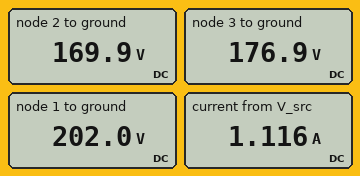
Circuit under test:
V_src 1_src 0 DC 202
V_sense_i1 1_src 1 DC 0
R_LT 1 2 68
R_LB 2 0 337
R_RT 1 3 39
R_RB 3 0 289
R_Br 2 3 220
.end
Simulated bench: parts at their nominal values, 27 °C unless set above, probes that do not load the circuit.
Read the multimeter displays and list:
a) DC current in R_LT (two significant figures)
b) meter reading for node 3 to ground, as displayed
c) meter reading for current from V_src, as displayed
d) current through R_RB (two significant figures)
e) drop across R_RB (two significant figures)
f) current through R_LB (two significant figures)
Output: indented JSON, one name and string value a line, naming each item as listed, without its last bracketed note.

{
  "DC current in R_LT": "470 mA",
  "meter reading for node 3 to ground, as displayed": "176.9 V",
  "meter reading for current from V_src, as displayed": "1.116 A",
  "current through R_RB": "610 mA",
  "drop across R_RB": "180 V",
  "current through R_LB": "500 mA"
}
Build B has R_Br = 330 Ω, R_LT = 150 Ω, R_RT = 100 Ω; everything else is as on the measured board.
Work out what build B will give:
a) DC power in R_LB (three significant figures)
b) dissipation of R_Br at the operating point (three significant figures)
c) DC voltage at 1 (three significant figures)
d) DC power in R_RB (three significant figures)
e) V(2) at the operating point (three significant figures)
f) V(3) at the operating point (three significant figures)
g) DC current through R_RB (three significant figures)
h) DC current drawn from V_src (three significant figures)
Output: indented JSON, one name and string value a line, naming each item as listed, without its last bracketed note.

{
  "DC power in R_LB": "59.7 W",
  "dissipation of R_Br at the operating point": "135 mW",
  "DC voltage at 1": "202 V",
  "DC power in R_RB": "76.4 W",
  "V(2) at the operating point": "142 V",
  "V(3) at the operating point": "149 V",
  "DC current through R_RB": "514 mA",
  "DC current drawn from V_src": "935 mA"
}
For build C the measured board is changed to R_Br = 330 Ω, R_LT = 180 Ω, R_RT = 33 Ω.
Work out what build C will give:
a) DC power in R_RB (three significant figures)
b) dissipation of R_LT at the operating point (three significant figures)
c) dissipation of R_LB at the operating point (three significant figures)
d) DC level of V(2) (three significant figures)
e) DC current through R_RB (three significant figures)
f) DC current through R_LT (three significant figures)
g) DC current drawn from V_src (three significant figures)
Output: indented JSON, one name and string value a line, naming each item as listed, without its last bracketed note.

{
  "DC power in R_RB": "110 W",
  "dissipation of R_LT at the operating point": "18.8 W",
  "dissipation of R_LB at the operating point": "61.4 W",
  "DC level of V(2)": "144 V",
  "DC current through R_RB": "617 mA",
  "DC current through R_LT": "323 mA",
  "DC current drawn from V_src": "1.04 A"
}
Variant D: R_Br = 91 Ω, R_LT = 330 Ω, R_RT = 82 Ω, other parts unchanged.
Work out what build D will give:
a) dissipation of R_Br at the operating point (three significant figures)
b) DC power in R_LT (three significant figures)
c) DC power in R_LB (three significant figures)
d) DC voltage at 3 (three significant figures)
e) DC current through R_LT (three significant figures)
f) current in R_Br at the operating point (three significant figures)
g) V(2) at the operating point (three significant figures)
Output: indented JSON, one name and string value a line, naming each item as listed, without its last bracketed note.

{
  "dissipation of R_Br at the operating point": "2.69 W",
  "DC power in R_LT": "15.4 W",
  "DC power in R_LB": "50.7 W",
  "DC voltage at 3": "146 V",
  "DC current through R_LT": "216 mA",
  "current in R_Br at the operating point": "172 mA",
  "V(2) at the operating point": "131 V"
}
